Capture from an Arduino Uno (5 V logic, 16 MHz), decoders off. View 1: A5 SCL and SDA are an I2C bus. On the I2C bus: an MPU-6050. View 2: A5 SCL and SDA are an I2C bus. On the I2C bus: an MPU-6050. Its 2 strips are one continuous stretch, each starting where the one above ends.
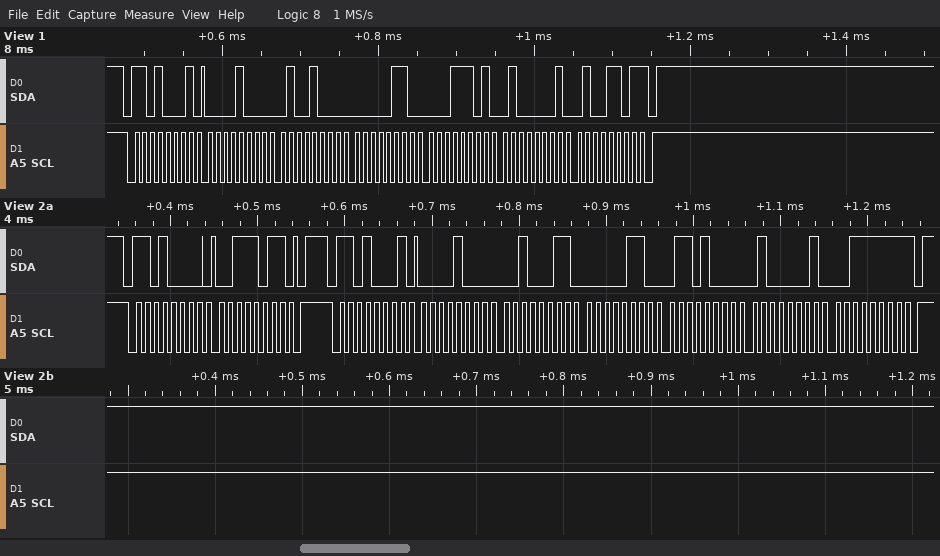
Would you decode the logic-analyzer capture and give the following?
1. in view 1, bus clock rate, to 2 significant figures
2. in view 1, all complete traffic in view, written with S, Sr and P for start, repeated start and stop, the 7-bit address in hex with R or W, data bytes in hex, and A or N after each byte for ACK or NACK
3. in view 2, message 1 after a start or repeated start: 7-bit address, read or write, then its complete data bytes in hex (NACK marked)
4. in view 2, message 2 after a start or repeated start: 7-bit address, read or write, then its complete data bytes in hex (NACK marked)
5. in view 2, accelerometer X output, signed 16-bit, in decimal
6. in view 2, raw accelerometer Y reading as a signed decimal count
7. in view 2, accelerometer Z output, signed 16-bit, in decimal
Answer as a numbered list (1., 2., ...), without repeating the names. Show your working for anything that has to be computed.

1. 100 kHz
2. S 68R A 08 A 48 A 06 A 1D A 41 A 4D N P
3. 0x68 write: 3B
4. 0x68 read: 08 23 06 68 41 3F NACK
5. 0x0823 = 2083
6. 0x0668 = 1640
7. 0x413F = 16703
